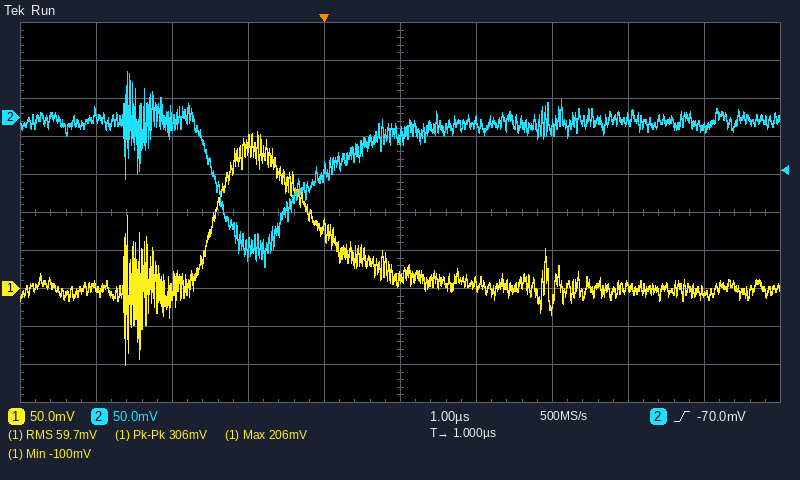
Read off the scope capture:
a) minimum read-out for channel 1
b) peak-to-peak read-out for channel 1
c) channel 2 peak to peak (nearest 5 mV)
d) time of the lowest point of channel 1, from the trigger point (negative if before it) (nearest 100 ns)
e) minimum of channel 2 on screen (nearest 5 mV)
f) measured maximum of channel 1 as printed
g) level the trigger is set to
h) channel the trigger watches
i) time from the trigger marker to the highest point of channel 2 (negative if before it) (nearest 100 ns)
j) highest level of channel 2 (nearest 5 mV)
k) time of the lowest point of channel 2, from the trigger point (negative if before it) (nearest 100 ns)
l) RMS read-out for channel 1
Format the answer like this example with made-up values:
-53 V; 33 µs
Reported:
-100 mV; 306 mV; 255 mV; -2.6 µs; -195 mV; 206 mV; -70.0 mV; channel 2; -2.6 µs; 60 mV; -800 ns; 59.7 mV
